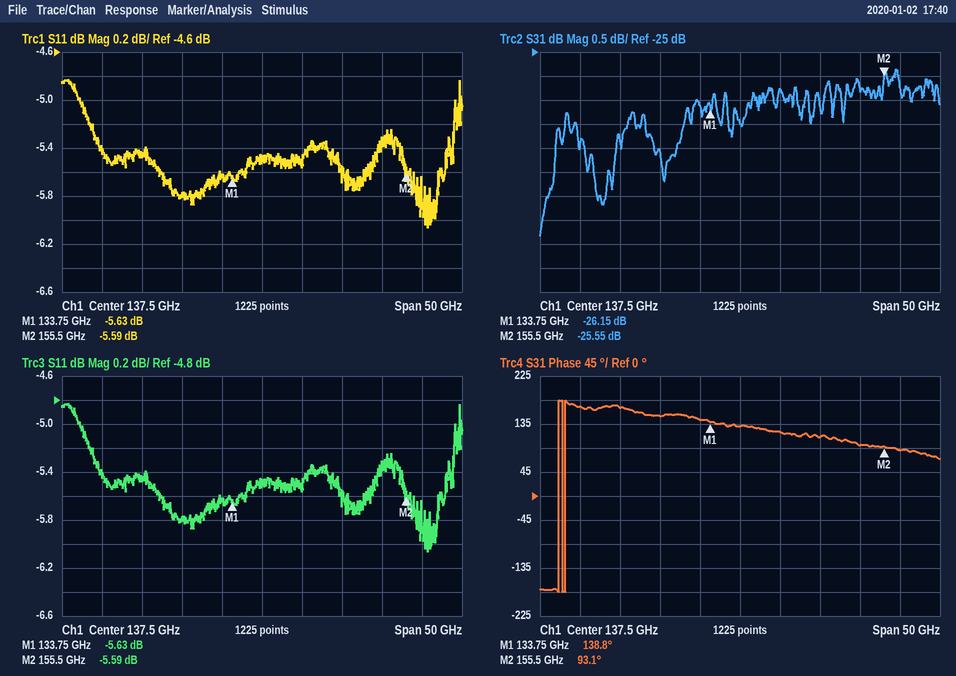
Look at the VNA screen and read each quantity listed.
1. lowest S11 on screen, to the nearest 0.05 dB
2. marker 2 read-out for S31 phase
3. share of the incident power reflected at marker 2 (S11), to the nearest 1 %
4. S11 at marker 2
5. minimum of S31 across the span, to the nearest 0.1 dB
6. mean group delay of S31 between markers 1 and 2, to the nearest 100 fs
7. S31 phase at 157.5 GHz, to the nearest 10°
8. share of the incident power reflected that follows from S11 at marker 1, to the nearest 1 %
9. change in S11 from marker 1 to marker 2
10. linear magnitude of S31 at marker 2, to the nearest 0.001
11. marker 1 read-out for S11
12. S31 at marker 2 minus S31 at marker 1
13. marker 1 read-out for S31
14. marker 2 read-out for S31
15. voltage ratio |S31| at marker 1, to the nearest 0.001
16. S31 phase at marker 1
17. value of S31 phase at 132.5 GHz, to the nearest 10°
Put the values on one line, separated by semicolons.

-6.05 dB; 93.1°; 28 %; -5.59 dB; -28.8 dB; 5.8 ps; 90°; 27 %; 0.04 dB; 0.053; -5.63 dB; 0.60 dB; -26.15 dB; -25.55 dB; 0.049; 138.8°; 140°
